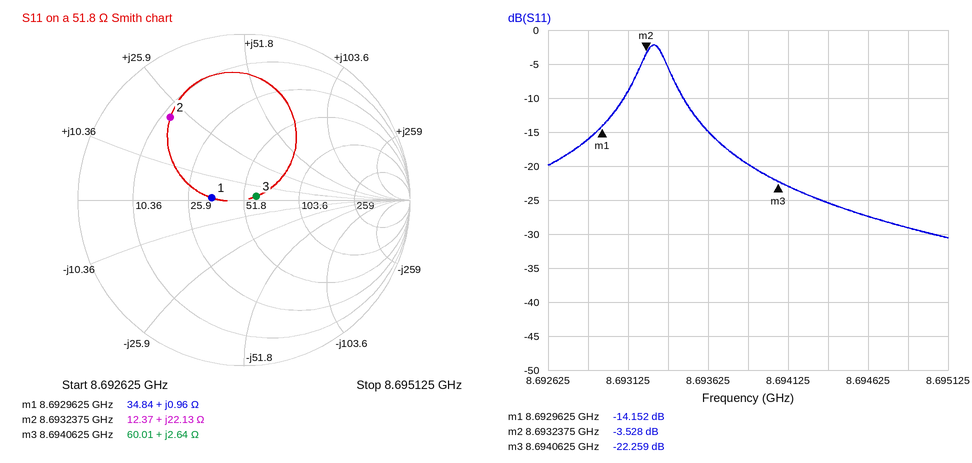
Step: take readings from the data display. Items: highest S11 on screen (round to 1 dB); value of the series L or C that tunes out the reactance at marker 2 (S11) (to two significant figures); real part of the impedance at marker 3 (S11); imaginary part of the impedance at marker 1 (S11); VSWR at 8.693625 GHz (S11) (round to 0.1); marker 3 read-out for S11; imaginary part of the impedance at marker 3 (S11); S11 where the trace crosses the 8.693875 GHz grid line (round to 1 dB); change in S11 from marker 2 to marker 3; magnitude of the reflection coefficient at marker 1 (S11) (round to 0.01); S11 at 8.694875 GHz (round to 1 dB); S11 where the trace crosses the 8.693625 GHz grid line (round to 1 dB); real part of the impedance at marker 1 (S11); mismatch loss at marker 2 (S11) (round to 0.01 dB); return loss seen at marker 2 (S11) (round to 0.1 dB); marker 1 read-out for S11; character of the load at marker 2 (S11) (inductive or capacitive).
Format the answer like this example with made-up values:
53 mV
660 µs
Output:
-2 dB
830 fF
60.01 Ω
+0.96 Ω
1.4
-22.259 dB
+2.64 Ω
-20 dB
-18.731 dB
0.20
-29 dB
-15 dB
34.84 Ω
2.55 dB
3.5 dB
-14.152 dB
inductive
